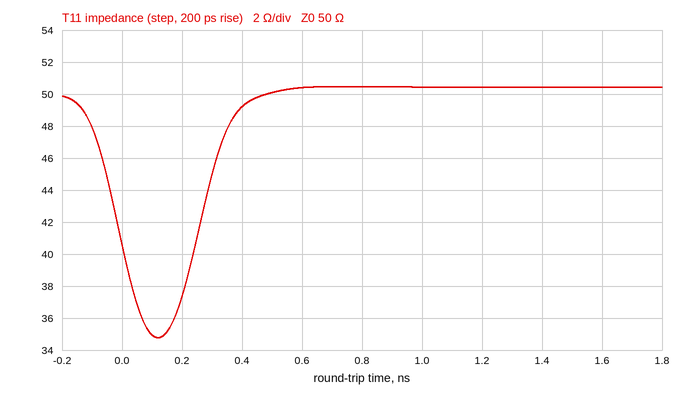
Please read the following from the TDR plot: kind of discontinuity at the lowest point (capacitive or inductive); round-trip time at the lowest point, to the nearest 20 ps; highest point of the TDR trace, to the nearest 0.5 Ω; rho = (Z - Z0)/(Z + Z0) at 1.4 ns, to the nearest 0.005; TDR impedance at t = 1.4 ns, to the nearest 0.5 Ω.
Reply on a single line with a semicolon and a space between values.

capacitive; 120 ps; 50.5 Ω; +0.005; 50.5 Ω
